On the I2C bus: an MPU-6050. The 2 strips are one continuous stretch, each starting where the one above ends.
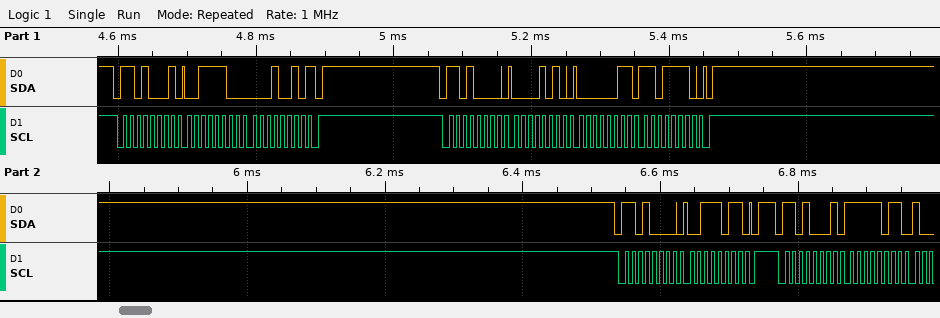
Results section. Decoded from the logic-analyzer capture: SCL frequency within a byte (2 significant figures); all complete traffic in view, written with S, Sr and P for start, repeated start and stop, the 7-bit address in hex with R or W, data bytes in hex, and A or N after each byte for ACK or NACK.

100 kHz
S 68R A 3C A 12 N P S 68W A 0A A 03 A DE A P S 68W A 3B A P S 68R A FB A
